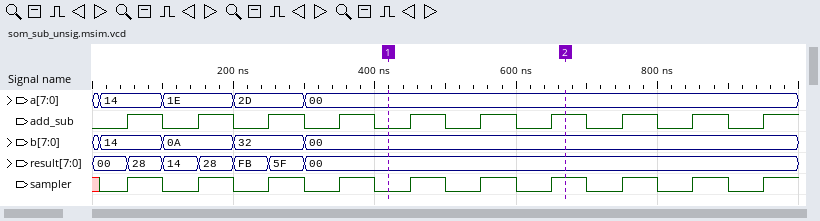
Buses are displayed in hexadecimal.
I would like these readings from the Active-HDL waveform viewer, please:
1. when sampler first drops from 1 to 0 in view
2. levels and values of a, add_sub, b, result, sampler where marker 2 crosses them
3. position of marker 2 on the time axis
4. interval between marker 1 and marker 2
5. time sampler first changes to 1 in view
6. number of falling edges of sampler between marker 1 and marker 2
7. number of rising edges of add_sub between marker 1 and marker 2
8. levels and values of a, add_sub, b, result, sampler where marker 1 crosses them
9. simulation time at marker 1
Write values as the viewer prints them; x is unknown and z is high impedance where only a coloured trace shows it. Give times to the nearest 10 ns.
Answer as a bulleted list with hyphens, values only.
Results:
- 100 ns
- a=00, add_sub=1, b=00, result=00, sampler=1
- 670 ns
- 250 ns
- 50 ns
- 2
- 3
- a=00, add_sub=0, b=00, result=00, sampler=0
- 420 ns
